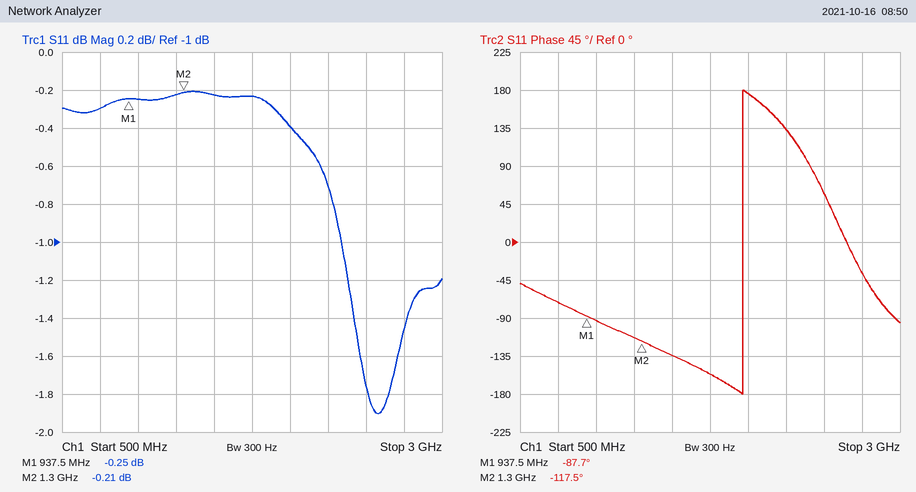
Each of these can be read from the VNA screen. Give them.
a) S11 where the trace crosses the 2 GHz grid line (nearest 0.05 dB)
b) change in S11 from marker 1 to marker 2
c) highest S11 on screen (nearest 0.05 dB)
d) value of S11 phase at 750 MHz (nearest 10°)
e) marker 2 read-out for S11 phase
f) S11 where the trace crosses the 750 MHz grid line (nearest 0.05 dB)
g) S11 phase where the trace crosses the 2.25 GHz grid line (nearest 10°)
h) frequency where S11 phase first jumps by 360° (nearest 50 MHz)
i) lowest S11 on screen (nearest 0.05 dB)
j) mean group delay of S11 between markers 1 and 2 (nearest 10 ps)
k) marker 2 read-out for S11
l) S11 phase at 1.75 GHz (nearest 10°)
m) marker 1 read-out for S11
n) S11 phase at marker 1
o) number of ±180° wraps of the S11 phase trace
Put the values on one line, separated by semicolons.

-0.40 dB; 0.04 dB; -0.20 dB; -70°; -117.5°; -0.30 dB; 130°; 1.95 GHz; -1.90 dB; 230 ps; -0.21 dB; -160°; -0.25 dB; -87.7°; 1
